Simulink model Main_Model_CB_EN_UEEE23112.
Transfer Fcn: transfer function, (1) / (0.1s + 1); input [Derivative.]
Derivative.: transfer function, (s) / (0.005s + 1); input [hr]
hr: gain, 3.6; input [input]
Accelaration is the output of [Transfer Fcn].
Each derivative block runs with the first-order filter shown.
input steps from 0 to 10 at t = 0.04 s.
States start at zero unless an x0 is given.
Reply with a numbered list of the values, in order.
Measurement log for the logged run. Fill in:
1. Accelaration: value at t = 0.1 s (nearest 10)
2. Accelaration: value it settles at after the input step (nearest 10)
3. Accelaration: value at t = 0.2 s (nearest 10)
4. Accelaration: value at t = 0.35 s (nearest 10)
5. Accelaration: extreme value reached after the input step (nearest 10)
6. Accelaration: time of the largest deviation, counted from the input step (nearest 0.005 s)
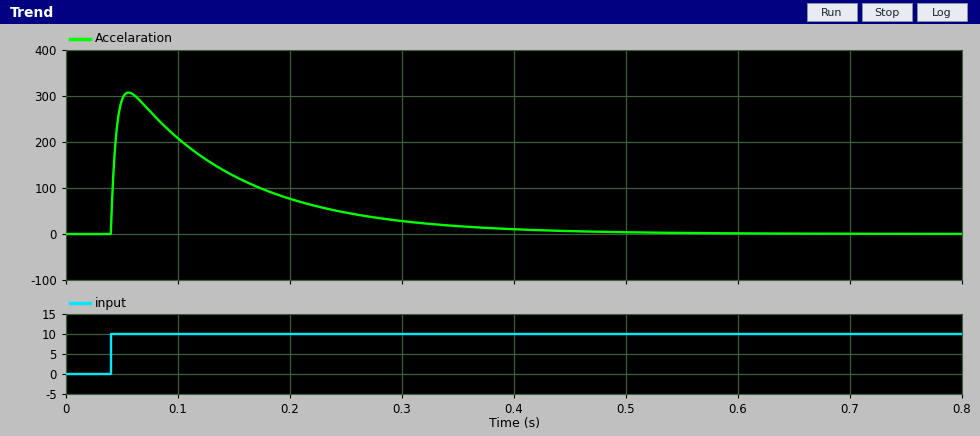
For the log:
1. 210
2. 0
3. 80
4. 20
5. 310
6. 0.015 s
